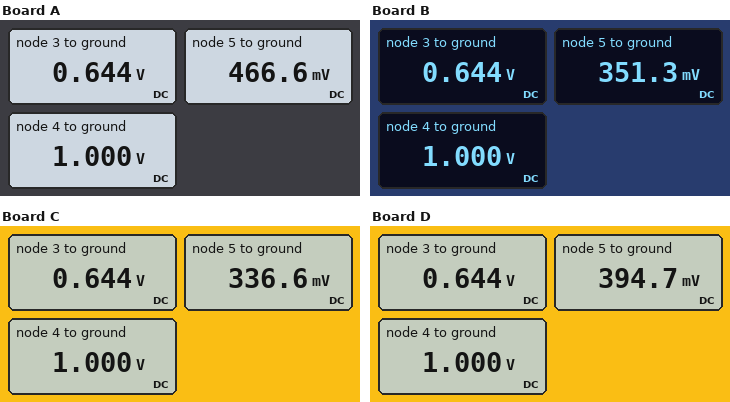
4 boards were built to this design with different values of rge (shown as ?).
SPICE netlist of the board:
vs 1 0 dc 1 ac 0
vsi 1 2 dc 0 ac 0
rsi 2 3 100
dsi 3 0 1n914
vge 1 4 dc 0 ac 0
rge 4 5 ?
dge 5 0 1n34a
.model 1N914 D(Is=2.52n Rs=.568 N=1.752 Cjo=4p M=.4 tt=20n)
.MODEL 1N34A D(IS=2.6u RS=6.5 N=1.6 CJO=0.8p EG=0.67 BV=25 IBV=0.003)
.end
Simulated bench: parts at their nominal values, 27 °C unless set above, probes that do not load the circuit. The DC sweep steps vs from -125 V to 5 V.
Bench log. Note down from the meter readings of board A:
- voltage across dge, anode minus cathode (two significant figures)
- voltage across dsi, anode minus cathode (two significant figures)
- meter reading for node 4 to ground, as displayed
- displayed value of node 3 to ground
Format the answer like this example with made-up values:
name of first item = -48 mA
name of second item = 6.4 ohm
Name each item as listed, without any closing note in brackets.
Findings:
voltage across dge, anode minus cathode = 470 mV
voltage across dsi, anode minus cathode = 640 mV
meter reading for node 4 to ground, as displayed = 1.000 V
displayed value of node 3 to ground = 0.644 V
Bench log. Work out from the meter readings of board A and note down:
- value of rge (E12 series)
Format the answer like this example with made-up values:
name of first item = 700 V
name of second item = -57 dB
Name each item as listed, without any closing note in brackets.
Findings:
value of rge = 33 Ω
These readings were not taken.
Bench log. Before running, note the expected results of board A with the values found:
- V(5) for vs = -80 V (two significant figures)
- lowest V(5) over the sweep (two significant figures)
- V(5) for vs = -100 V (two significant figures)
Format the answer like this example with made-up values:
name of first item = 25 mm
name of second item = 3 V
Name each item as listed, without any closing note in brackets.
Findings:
V(5) for vs = -80 V = -34 V
lowest V(5) over the sweep = -42 V
V(5) for vs = -100 V = -38 V
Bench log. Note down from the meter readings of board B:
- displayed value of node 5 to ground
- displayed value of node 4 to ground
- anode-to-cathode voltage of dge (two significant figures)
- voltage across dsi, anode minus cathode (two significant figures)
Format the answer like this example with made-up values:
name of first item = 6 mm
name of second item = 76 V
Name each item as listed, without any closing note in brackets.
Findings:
displayed value of node 5 to ground = 351.3 mV
displayed value of node 4 to ground = 1.000 V
anode-to-cathode voltage of dge = 350 mV
voltage across dsi, anode minus cathode = 640 mV
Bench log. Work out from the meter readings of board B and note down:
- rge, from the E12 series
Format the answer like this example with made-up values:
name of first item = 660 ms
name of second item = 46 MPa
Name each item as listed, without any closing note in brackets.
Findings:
rge, from the E12 series = 120 Ω
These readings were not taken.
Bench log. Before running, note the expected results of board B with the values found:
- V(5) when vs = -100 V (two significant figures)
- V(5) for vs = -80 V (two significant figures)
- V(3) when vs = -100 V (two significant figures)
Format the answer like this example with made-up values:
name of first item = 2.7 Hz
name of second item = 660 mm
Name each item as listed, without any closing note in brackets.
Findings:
V(5) when vs = -100 V = -29 V
V(5) for vs = -80 V = -28 V
V(3) when vs = -100 V = -100 V
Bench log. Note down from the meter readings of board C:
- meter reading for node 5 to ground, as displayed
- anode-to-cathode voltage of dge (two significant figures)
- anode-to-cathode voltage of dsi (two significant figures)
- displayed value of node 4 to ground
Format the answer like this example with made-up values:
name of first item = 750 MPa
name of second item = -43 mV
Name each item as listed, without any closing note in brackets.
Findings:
meter reading for node 5 to ground, as displayed = 336.6 mV
anode-to-cathode voltage of dge = 340 mV
anode-to-cathode voltage of dsi = 640 mV
displayed value of node 4 to ground = 1.000 V
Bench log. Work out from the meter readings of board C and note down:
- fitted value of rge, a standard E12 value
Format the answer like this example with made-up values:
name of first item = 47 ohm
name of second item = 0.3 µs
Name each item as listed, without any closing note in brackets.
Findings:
fitted value of rge, a standard E12 value = 150 Ω
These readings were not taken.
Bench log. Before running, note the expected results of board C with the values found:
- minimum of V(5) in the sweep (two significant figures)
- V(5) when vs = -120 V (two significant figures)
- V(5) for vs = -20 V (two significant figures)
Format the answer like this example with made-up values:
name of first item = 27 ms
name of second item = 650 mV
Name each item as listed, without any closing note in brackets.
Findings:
minimum of V(5) in the sweep = -29 V
V(5) when vs = -120 V = -29 V
V(5) for vs = -20 V = -20 V
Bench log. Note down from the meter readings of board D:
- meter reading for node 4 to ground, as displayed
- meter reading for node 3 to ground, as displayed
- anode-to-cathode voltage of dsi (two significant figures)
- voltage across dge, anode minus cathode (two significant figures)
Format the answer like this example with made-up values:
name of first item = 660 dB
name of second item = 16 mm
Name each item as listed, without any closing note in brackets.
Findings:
meter reading for node 4 to ground, as displayed = 1.000 V
meter reading for node 3 to ground, as displayed = 0.644 V
anode-to-cathode voltage of dsi = 640 mV
voltage across dge, anode minus cathode = 390 mV
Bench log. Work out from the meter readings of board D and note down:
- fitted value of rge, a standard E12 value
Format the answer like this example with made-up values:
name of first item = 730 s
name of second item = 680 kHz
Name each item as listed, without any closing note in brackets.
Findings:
fitted value of rge, a standard E12 value = 68 Ω
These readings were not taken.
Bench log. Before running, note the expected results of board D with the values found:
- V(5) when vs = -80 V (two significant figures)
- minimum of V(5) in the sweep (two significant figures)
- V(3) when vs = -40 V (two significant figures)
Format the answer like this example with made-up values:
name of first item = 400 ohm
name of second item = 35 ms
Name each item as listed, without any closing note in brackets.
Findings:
V(5) when vs = -80 V = -30 V
minimum of V(5) in the sweep = -34 V
V(3) when vs = -40 V = -40 V
